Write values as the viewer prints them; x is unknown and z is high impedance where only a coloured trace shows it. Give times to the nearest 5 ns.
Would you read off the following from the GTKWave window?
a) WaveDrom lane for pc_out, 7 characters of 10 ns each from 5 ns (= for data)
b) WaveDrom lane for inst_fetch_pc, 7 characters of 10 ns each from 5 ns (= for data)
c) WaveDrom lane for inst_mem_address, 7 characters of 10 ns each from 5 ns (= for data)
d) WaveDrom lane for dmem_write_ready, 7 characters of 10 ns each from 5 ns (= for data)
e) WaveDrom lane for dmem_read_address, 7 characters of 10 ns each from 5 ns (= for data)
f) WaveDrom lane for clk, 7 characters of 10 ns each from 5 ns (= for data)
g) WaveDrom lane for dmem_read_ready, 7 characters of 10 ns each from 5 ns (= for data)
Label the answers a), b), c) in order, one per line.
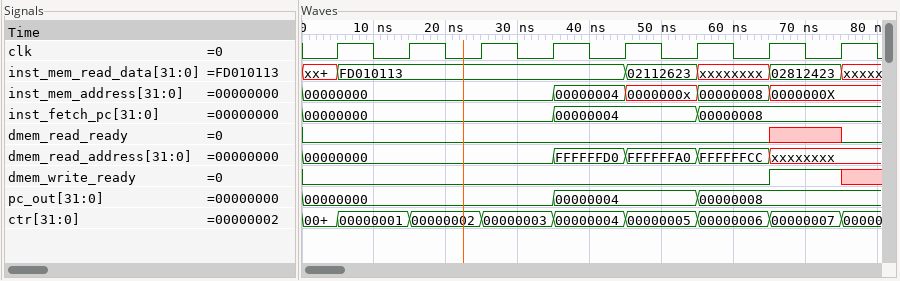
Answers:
a) {name: 'pc_out', wave: '=..=.=.', data: '00000000 00000004 00000008'}
b) {name: 'inst_fetch_pc', wave: '=..=.=.', data: '00000000 00000004 00000008'}
c) {name: 'inst_mem_address', wave: '=..====', data: '00000000 00000004 0000000x 00000008 0000000X'}
d) {name: 'dmem_write_ready', wave: '0.....1'}
e) {name: 'dmem_read_address', wave: '=..===x', data: '00000000 FFFFFFD0 FFFFFFA0 FFFFFFCC'}
f) {name: 'clk', wave: 'p......'}
g) {name: 'dmem_read_ready', wave: '0.....x'}
